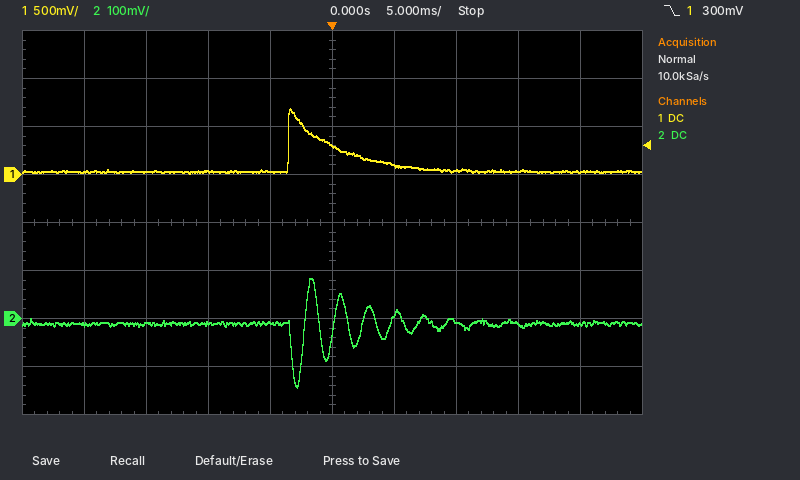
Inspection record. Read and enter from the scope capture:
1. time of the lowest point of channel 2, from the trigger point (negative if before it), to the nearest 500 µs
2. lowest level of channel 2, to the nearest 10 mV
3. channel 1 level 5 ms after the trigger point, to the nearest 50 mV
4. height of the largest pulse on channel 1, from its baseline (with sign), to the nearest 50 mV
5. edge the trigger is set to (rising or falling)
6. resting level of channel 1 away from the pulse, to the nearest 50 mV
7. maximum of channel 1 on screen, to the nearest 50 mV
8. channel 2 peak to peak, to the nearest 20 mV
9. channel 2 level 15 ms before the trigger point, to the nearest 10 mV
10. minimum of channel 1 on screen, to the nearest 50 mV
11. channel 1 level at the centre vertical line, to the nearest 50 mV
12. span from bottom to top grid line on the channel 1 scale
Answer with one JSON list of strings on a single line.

["-3.0 ms", "-140 mV", "100 mV", "+650 mV", "falling", "50 mV", "700 mV", "220 mV", "-10 mV", "0 mV", "300 mV", "4 V"]
